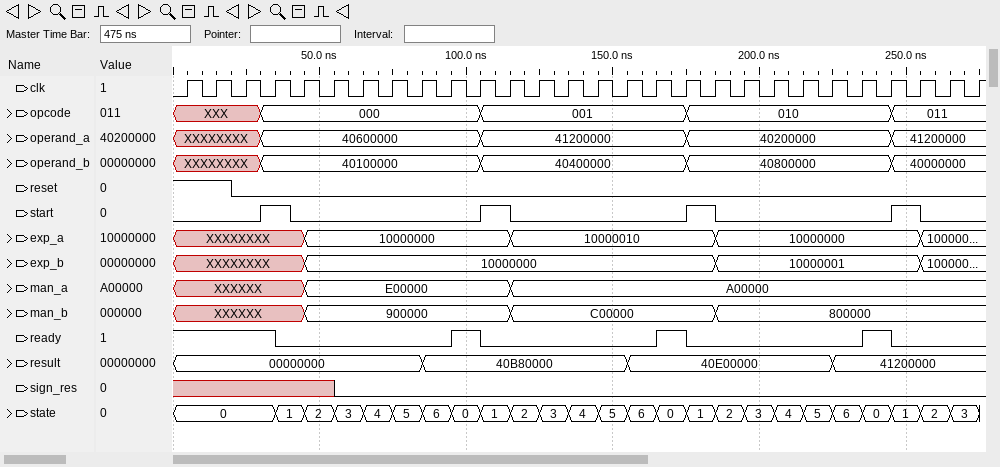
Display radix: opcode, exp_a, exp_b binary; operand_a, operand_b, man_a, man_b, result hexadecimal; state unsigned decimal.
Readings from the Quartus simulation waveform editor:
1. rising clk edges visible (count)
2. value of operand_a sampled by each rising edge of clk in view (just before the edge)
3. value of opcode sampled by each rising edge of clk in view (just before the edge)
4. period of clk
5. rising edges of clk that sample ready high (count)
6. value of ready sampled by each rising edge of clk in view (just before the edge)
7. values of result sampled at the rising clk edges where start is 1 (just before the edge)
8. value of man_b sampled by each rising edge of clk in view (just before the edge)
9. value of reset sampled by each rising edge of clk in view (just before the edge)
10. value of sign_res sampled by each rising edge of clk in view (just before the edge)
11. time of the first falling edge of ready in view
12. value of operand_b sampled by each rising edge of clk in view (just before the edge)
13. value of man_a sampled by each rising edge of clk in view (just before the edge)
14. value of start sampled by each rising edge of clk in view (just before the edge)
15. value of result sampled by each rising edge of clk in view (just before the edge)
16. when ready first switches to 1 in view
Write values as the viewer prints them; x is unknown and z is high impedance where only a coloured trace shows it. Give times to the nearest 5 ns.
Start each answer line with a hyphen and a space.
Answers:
- 28
- XXXXXXXX, XXXXXXXX, XXXXXXXX, 40600000, 40600000, 40600000, 40600000, 40600000, 40600000, 40600000, 40600000, 41200000, 41200000, 41200000, 41200000, 41200000, 41200000, 41200000, 40200000, 40200000, 40200000, 40200000, 40200000, 40200000, 40200000, 41200000, 41200000, 41200000
- XXX, XXX, XXX, 000, 000, 000, 000, 000, 000, 000, 000, 001, 001, 001, 001, 001, 001, 001, 010, 010, 010, 010, 010, 010, 010, 011, 011, 011
- 10 ns
- 7
- 1 1 1 1 0 0 0 0 0 0 1 0 0 0 0 0 0 1 0 0 0 0 0 0 1 0 0 0
- 00000000, 40B80000, 40E00000, 41200000
- XXXXXX, XXXXXX, XXXXXX, XXXXXX, XXXXXX, 900000, 900000, 900000, 900000, 900000, 900000, 900000, C00000, C00000, C00000, C00000, C00000, C00000, C00000, 800000, 800000, 800000, 800000, 800000, 800000, 800000, 800000, 800000
- 1 1 0 0 0 0 0 0 0 0 0 0 0 0 0 0 0 0 0 0 0 0 0 0 0 0 0 0
- x x x x x x 0 0 0 0 0 0 0 0 0 0 0 0 0 0 0 0 0 0 0 0 0 0
- 35 ns
- XXXXXXXX, XXXXXXXX, XXXXXXXX, 40100000, 40100000, 40100000, 40100000, 40100000, 40100000, 40100000, 40100000, 40400000, 40400000, 40400000, 40400000, 40400000, 40400000, 40400000, 40800000, 40800000, 40800000, 40800000, 40800000, 40800000, 40800000, 40000000, 40000000, 40000000
- XXXXXX, XXXXXX, XXXXXX, XXXXXX, XXXXXX, E00000, E00000, E00000, E00000, E00000, E00000, E00000, A00000, A00000, A00000, A00000, A00000, A00000, A00000, A00000, A00000, A00000, A00000, A00000, A00000, A00000, A00000, A00000
- 0 0 0 1 0 0 0 0 0 0 0 1 0 0 0 0 0 0 1 0 0 0 0 0 0 1 0 0
- 00000000, 00000000, 00000000, 00000000, 00000000, 00000000, 00000000, 00000000, 00000000, 40B80000, 40B80000, 40B80000, 40B80000, 40B80000, 40B80000, 40B80000, 40E00000, 40E00000, 40E00000, 40E00000, 40E00000, 40E00000, 40E00000, 41200000, 41200000, 41200000, 41200000, 41200000
- 95 ns
